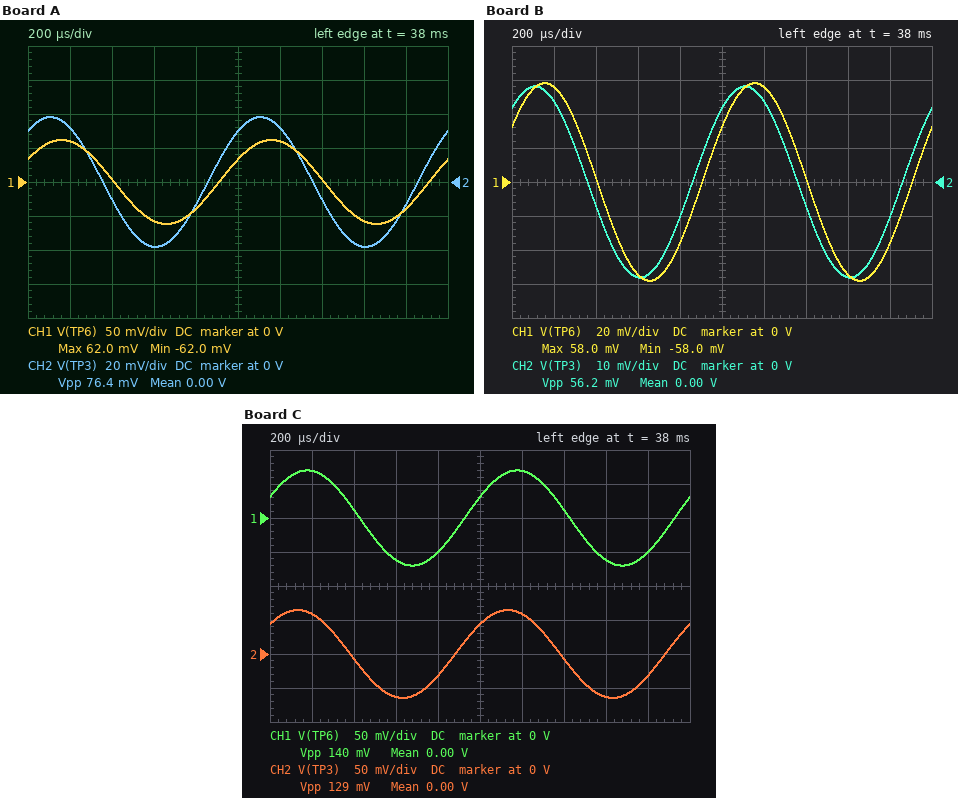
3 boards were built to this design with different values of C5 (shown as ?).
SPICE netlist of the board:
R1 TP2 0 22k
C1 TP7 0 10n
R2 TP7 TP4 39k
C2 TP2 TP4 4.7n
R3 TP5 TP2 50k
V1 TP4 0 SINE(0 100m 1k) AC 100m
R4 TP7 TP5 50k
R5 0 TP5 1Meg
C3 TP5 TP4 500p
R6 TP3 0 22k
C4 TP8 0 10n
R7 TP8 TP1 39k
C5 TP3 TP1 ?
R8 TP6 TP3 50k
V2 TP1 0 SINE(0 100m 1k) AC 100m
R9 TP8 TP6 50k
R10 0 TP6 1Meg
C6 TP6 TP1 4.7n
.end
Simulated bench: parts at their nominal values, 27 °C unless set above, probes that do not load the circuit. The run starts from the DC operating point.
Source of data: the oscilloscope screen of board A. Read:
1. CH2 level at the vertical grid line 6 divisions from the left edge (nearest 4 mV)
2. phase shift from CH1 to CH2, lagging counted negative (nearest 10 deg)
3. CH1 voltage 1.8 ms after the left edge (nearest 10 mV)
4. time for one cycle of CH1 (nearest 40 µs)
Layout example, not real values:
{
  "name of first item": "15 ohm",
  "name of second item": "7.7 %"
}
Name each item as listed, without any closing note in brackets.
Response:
{
  "CH2 level at the vertical grid line 6 divisions from the left edge": "32 mV",
  "phase shift from CH1 to CH2, lagging counted negative": "20 deg",
  "CH1 voltage 1.8 ms after the left edge": "-40 mV",
  "time for one cycle of CH1": "1.00 ms"
}
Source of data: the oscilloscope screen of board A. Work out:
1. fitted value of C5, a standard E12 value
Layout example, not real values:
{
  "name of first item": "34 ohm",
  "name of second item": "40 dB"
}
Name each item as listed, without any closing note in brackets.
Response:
{
  "fitted value of C5, a standard E12 value": "2.7 nF"
}
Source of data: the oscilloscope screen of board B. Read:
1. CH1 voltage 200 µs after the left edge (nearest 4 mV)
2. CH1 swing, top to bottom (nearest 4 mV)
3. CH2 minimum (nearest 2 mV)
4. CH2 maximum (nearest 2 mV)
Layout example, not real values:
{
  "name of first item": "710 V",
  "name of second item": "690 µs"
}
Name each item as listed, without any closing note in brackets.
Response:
{
  "CH1 voltage 200 µs after the left edge": "56 mV",
  "CH1 swing, top to bottom": "116 mV",
  "CH2 minimum": "-28 mV",
  "CH2 maximum": "28 mV"
}
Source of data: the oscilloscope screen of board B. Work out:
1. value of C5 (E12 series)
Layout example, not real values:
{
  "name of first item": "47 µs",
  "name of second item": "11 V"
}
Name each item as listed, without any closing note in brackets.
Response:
{
  "value of C5": "1.5 nF"
}
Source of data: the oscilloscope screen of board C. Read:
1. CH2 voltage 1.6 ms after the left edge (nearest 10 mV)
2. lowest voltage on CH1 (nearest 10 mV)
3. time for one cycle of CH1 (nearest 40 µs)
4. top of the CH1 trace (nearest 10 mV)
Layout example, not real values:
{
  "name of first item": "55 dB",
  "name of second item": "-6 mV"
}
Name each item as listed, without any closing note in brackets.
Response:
{
  "CH2 voltage 1.6 ms after the left edge": "-60 mV",
  "lowest voltage on CH1": "-70 mV",
  "time for one cycle of CH1": "1.00 ms",
  "top of the CH1 trace": "70 mV"
}
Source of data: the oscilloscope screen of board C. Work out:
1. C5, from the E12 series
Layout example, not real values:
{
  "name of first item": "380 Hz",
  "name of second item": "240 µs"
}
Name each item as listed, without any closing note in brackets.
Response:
{
  "C5, from the E12 series": "6.8 nF"
}
